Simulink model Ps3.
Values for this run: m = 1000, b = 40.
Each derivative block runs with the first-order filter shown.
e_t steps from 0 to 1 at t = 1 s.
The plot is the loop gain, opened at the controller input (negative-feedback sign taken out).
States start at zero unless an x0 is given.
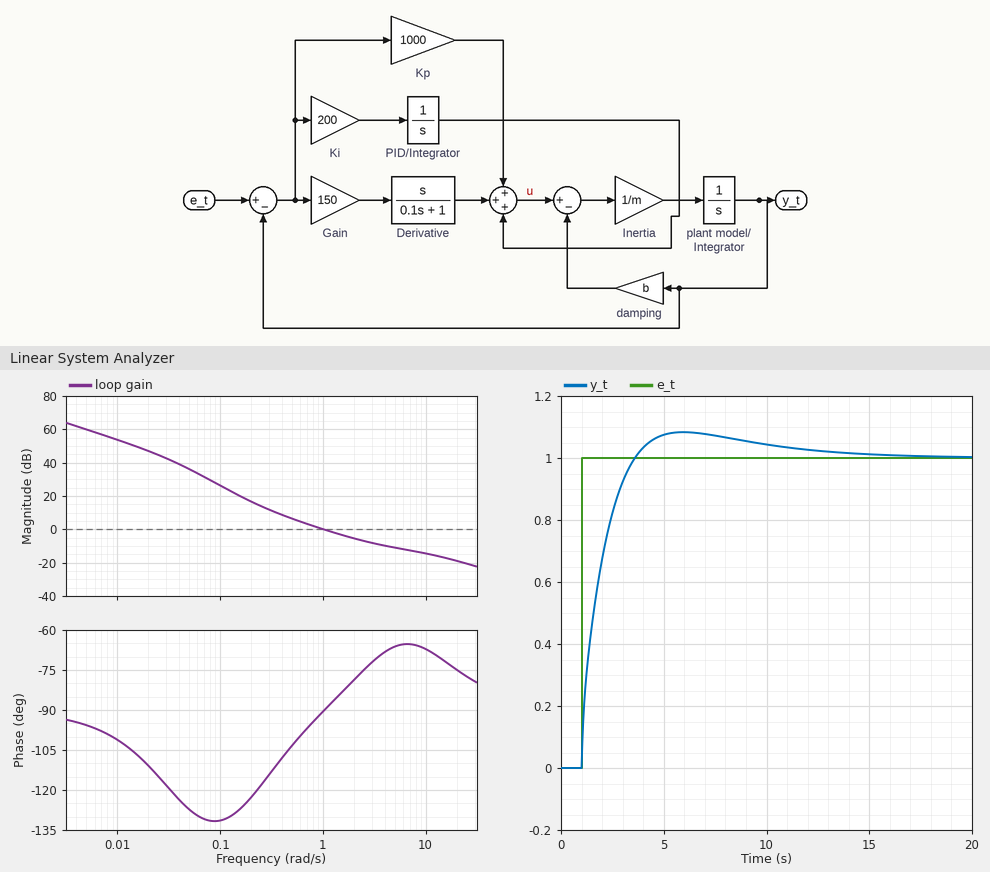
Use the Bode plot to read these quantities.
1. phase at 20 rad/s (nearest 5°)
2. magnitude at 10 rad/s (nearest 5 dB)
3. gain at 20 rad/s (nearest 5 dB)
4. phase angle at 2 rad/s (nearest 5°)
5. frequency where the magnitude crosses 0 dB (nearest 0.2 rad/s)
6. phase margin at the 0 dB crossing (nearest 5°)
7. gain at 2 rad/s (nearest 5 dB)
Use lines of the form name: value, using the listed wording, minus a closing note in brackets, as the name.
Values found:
phase at 20 rad/s: -75°
magnitude at 10 rad/s: -15 dB
gain at 20 rad/s: -20 dB
phase angle at 2 rad/s: -80°
frequency where the magnitude crosses 0 dB: 1.0 rad/s
phase margin at the 0 dB crossing: 90°
gain at 2 rad/s: -5 dB
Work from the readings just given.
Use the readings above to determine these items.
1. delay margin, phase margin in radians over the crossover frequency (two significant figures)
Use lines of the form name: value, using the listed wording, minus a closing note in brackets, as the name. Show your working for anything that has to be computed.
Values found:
delay margin, phase margin in radians over the crossover frequency: 90 × π / 180 / 1 = 1.6 s
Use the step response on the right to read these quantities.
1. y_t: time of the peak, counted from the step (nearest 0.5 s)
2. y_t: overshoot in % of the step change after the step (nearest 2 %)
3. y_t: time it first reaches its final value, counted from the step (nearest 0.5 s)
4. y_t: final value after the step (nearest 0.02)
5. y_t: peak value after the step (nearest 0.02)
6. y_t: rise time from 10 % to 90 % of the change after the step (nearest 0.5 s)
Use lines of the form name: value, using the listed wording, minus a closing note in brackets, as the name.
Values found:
y_t: time of the peak, counted from the step: 5.0 s
y_t: overshoot in % of the step change after the step: 8 %
y_t: time it first reaches its final value, counted from the step: 2.5 s
y_t: final value after the step: 1.00
y_t: peak value after the step: 1.08
y_t: rise time from 10 % to 90 % of the change after the step: 2.0 s
